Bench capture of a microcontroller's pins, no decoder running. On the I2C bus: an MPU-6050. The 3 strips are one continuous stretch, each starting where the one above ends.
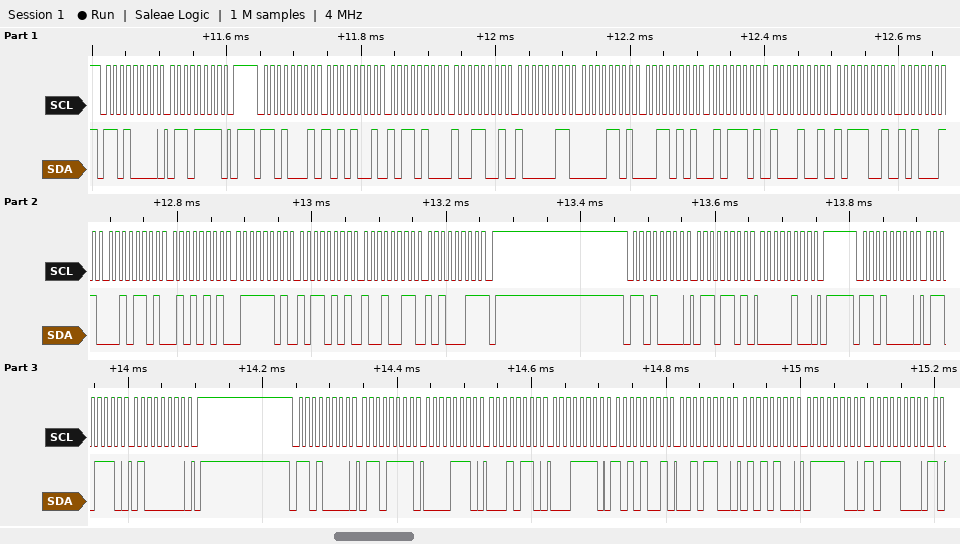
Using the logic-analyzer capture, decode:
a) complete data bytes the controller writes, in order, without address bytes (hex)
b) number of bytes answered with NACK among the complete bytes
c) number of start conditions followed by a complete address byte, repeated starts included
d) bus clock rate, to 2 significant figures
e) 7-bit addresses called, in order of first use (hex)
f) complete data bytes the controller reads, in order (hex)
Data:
6F 6D 04 6E 40 6F 0E 16 1E A9 2C 54 7C B8
1
5
100 kHz
0x68
A9 B4 99 83 0D 35 5D 89 B9 A3 2D 55 7D B5 93 A3
